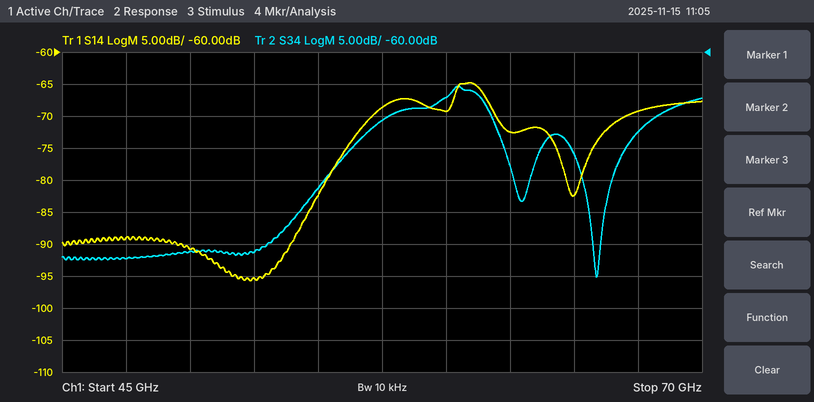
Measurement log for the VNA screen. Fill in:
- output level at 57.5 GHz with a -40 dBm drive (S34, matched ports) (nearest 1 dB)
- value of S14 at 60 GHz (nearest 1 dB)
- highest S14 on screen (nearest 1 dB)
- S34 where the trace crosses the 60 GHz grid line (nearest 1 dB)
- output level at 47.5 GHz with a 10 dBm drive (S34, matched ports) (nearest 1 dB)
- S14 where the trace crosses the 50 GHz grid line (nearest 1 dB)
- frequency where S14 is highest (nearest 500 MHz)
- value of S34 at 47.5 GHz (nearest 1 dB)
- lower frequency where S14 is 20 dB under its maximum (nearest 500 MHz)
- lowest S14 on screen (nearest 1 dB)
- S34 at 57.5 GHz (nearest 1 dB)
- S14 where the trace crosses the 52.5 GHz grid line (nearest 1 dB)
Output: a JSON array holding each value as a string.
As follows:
["-111 dBm", "-69 dB", "-65 dB", "-67 dB", "-82 dBm", "-91 dB", "61.0 GHz", "-92 dB", "54.5 GHz", "-96 dB", "-71 dB", "-95 dB"]
